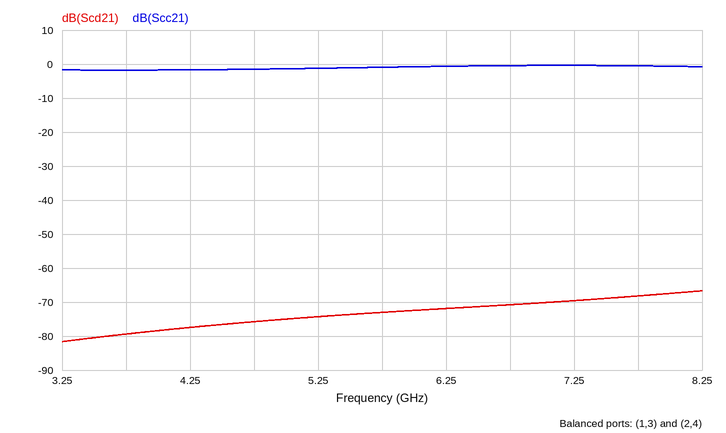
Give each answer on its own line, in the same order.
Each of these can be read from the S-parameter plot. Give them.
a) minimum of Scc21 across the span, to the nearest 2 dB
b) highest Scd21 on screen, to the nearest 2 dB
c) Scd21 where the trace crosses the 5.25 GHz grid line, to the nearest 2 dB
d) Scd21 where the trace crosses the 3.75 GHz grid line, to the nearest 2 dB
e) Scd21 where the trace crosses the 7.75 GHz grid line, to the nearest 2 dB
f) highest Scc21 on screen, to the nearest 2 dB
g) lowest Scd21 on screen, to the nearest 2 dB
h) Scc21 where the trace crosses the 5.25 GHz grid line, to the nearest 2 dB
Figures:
-2 dB
-66 dB
-74 dB
-80 dB
-68 dB
0 dB
-82 dB
-2 dB
